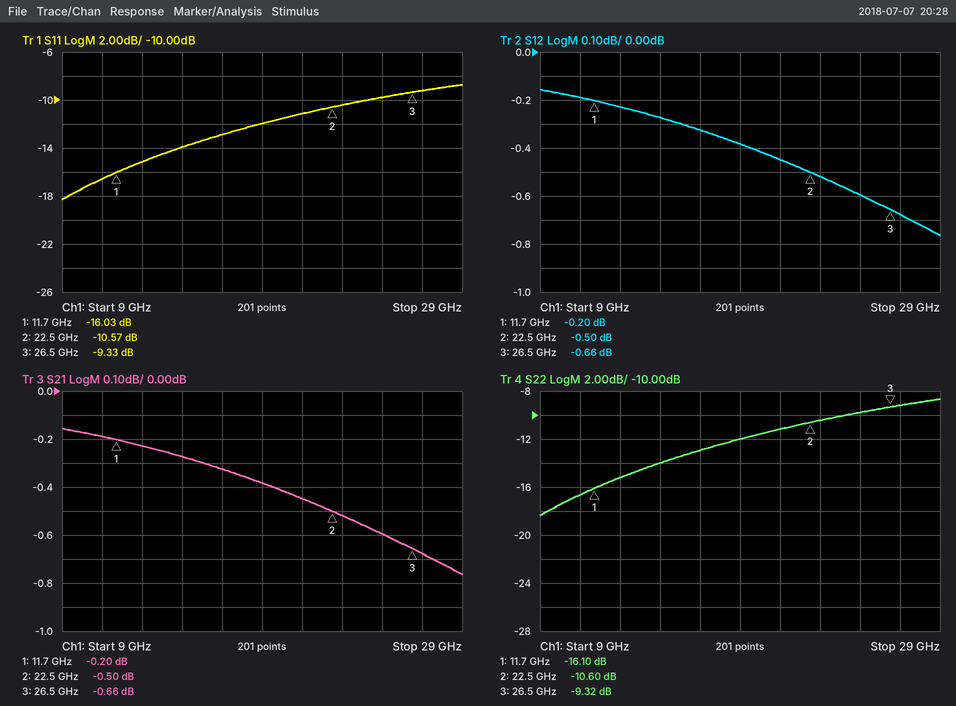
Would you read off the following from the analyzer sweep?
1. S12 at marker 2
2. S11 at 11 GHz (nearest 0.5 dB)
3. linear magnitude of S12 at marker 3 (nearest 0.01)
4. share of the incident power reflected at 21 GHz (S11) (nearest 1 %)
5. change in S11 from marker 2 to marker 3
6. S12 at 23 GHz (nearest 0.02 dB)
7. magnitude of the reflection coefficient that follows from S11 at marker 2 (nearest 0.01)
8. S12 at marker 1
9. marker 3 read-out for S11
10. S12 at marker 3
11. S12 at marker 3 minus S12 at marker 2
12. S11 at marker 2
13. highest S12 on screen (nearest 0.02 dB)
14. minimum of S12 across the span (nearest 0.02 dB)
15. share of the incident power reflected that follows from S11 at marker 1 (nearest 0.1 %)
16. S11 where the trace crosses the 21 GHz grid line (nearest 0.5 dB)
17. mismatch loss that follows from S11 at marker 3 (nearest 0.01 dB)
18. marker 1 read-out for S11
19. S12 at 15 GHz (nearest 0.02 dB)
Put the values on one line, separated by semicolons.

-0.50 dB; -16.5 dB; 0.93; 8 %; 1.24 dB; -0.52 dB; 0.30; -0.20 dB; -9.33 dB; -0.66 dB; -0.16 dB; -10.57 dB; -0.16 dB; -0.76 dB; 2.5 %; -11.0 dB; 0.54 dB; -16.03 dB; -0.28 dB
